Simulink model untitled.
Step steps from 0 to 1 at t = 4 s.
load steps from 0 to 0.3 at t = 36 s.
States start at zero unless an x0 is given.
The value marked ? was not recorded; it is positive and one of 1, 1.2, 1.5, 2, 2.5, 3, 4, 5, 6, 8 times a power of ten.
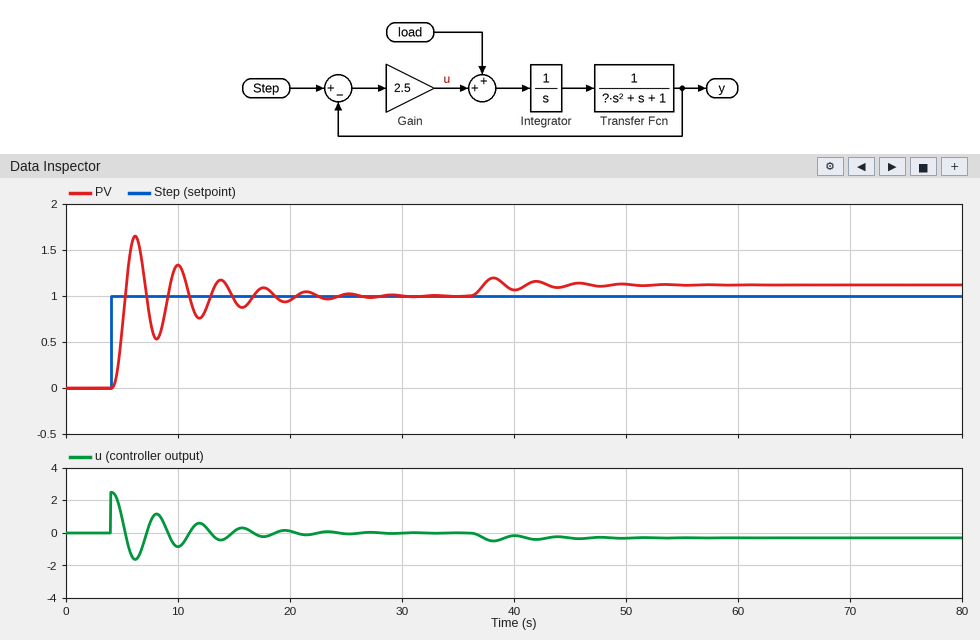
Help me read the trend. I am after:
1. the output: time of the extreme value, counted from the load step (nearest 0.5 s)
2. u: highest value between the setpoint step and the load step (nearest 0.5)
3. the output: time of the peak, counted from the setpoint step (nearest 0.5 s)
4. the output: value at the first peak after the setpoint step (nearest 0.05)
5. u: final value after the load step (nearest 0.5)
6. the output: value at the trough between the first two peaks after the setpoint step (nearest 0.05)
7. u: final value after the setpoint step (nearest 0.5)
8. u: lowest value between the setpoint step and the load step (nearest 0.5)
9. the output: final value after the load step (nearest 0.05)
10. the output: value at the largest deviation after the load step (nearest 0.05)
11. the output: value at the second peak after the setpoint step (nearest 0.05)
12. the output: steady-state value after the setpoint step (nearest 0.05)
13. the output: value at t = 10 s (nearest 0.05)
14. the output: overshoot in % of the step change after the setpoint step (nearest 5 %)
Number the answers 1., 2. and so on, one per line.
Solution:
1. 2.0 s
2. 2.5
3. 2.0 s
4. 1.65
5. -0.5
6. 0.55
7. 0.0
8. -1.5
9. 1.10
10. 1.20
11. 1.35
12. 1.00
13. 1.35
14. 65 %
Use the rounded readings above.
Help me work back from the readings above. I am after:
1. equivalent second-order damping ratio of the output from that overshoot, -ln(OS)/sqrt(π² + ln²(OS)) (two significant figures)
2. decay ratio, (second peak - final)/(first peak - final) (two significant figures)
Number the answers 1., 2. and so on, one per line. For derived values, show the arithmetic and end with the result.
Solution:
1. ln(0.65) = -0.431; 0.431 / sqrt(9.870 + 0.186) = 0.14
2. (1.35 - 1) / (1.65 - 1) = 0.54
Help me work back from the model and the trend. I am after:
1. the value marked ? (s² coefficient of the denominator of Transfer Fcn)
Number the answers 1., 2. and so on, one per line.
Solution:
1. 0.25
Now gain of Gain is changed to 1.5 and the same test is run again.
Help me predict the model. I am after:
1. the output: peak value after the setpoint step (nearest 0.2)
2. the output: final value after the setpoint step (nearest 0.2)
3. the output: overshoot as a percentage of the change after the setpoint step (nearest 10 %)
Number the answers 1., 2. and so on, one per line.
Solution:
1. 1.4
2. 1.0
3. 40 %
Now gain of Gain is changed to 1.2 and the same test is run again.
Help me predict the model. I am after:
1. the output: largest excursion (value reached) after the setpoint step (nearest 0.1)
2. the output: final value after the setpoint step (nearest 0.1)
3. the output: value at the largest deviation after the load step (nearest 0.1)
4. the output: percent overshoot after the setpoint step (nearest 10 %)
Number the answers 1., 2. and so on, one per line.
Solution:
1. 1.3
2. 1.0
3. 1.3
4. 30 %
